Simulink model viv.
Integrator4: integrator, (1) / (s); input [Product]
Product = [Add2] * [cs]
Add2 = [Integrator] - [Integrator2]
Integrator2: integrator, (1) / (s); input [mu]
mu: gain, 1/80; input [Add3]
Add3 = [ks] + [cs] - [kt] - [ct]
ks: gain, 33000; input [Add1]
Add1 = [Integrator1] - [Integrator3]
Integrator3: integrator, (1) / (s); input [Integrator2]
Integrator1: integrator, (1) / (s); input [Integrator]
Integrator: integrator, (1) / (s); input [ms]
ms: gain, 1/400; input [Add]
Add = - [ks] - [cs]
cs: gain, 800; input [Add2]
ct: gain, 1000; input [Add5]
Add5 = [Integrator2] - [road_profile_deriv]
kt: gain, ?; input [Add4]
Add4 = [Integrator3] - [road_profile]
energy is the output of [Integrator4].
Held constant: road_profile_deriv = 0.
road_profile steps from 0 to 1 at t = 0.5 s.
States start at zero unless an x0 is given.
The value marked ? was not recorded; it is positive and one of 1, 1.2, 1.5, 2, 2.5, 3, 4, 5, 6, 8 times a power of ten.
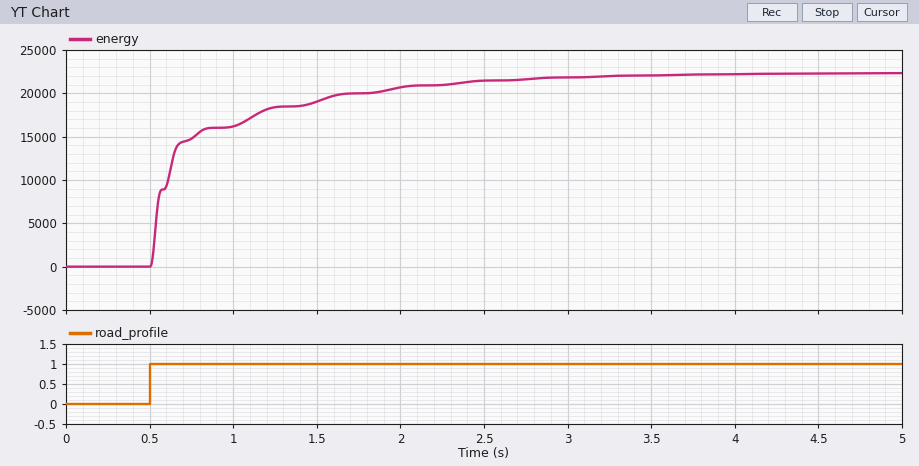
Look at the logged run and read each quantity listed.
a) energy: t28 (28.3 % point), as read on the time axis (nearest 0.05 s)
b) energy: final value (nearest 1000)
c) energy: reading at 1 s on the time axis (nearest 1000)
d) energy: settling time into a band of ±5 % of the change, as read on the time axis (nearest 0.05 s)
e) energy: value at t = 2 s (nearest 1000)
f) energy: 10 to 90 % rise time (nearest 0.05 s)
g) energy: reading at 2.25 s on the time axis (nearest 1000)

0.55 s
22000
16000
2.40 s
21000
1.35 s
21000
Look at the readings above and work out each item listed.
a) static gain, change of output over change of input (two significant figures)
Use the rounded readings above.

22000
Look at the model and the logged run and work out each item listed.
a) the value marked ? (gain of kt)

80000
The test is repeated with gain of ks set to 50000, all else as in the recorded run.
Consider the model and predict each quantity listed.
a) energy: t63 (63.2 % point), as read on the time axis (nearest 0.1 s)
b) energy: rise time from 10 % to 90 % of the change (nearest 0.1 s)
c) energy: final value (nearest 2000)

0.8 s
1.5 s
22000
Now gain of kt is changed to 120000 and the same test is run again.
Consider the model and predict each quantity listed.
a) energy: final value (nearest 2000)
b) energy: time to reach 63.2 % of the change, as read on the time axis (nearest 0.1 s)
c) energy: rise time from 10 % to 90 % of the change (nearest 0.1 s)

34000
0.6 s
1.0 s
